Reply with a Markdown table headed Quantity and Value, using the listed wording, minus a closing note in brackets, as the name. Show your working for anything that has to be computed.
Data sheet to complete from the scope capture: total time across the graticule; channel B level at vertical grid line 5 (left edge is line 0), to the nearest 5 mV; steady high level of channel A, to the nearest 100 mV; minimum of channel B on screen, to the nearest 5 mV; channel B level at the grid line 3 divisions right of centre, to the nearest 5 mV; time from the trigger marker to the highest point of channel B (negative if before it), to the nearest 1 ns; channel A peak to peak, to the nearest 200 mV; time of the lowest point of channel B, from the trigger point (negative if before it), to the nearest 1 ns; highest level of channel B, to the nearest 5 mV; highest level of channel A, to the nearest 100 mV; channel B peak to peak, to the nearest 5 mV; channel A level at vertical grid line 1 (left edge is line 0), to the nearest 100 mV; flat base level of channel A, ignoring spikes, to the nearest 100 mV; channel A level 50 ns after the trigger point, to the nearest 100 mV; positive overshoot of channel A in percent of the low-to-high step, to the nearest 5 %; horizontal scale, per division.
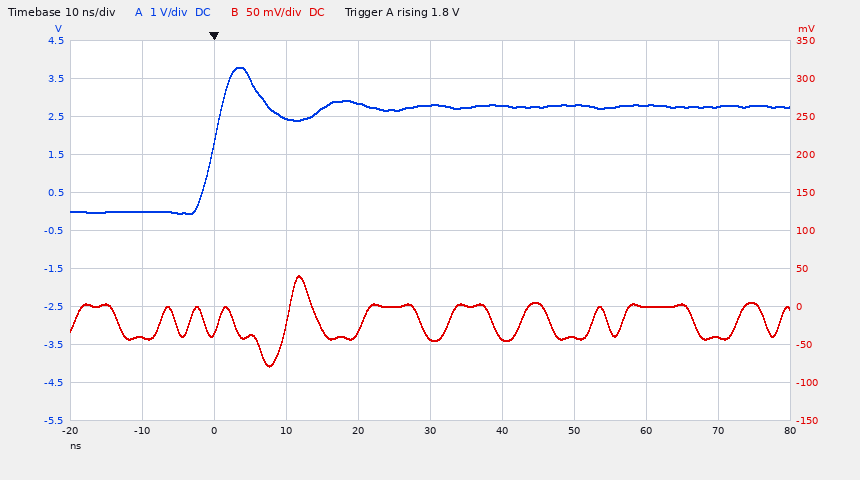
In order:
| Quantity | Value |
|---|---|
| total time across the graticule | 100 ns |
| channel B level at vertical grid line 5 (left edge is line 0), to the nearest 5 mV | -40 mV |
| steady high level of channel A, to the nearest 100 mV | 2.8 V |
| minimum of channel B on screen, to the nearest 5 mV | -80 mV |
| channel B level at the grid line 3 divisions right of centre, to the nearest 5 mV | 0 mV |
| time from the trigger marker to the highest point of channel B (negative if before it), to the nearest 1 ns | +12 ns |
| channel A peak to peak, to the nearest 200 mV | 3.8 V |
| time of the lowest point of channel B, from the trigger point (negative if before it), to the nearest 1 ns | +8 ns |
| highest level of channel B, to the nearest 5 mV | 40 mV |
| highest level of channel A, to the nearest 100 mV | 3.8 V |
| channel B peak to peak, to the nearest 5 mV | 40 mV − (-80 mV) = 120 mV |
| channel A level at vertical grid line 1 (left edge is line 0), to the nearest 100 mV | 0.0 V |
| flat base level of channel A, ignoring spikes, to the nearest 100 mV | 0.0 V |
| channel A level 50 ns after the trigger point, to the nearest 100 mV | 2.8 V |
| positive overshoot of channel A in percent of the low-to-high step, to the nearest 5 % | 35 % |
| horizontal scale, per division | 10 ns |
